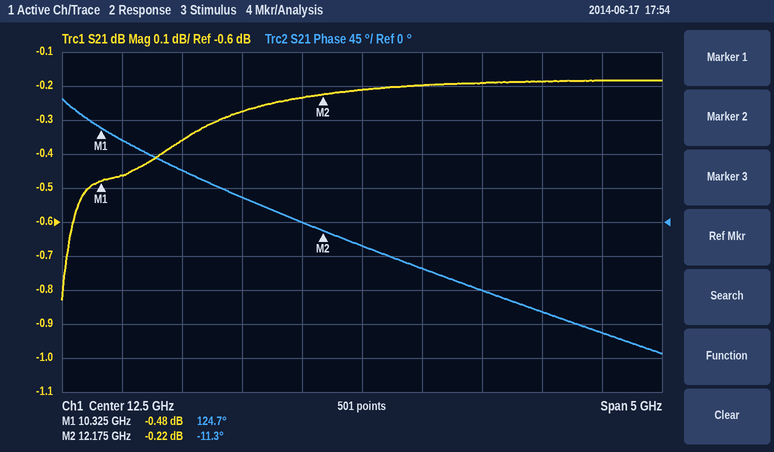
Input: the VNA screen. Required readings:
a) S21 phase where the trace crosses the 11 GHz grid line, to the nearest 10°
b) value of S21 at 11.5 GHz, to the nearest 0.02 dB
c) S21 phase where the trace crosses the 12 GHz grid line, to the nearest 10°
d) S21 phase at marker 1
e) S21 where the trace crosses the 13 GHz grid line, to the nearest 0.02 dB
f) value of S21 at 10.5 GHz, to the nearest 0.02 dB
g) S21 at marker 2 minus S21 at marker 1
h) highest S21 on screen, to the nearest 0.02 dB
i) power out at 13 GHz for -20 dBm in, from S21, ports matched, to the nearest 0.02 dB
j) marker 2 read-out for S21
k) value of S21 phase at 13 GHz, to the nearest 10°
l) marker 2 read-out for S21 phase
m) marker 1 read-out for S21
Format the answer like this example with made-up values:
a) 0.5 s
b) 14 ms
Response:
a) 70°
b) -0.28 dB
c) 0°
d) 124.7°
e) -0.20 dB
f) -0.46 dB
g) 0.26 dB
h) -0.18 dB
i) -20.20 dBm
j) -0.22 dB
k) -60°
l) -11.3°
m) -0.48 dB
